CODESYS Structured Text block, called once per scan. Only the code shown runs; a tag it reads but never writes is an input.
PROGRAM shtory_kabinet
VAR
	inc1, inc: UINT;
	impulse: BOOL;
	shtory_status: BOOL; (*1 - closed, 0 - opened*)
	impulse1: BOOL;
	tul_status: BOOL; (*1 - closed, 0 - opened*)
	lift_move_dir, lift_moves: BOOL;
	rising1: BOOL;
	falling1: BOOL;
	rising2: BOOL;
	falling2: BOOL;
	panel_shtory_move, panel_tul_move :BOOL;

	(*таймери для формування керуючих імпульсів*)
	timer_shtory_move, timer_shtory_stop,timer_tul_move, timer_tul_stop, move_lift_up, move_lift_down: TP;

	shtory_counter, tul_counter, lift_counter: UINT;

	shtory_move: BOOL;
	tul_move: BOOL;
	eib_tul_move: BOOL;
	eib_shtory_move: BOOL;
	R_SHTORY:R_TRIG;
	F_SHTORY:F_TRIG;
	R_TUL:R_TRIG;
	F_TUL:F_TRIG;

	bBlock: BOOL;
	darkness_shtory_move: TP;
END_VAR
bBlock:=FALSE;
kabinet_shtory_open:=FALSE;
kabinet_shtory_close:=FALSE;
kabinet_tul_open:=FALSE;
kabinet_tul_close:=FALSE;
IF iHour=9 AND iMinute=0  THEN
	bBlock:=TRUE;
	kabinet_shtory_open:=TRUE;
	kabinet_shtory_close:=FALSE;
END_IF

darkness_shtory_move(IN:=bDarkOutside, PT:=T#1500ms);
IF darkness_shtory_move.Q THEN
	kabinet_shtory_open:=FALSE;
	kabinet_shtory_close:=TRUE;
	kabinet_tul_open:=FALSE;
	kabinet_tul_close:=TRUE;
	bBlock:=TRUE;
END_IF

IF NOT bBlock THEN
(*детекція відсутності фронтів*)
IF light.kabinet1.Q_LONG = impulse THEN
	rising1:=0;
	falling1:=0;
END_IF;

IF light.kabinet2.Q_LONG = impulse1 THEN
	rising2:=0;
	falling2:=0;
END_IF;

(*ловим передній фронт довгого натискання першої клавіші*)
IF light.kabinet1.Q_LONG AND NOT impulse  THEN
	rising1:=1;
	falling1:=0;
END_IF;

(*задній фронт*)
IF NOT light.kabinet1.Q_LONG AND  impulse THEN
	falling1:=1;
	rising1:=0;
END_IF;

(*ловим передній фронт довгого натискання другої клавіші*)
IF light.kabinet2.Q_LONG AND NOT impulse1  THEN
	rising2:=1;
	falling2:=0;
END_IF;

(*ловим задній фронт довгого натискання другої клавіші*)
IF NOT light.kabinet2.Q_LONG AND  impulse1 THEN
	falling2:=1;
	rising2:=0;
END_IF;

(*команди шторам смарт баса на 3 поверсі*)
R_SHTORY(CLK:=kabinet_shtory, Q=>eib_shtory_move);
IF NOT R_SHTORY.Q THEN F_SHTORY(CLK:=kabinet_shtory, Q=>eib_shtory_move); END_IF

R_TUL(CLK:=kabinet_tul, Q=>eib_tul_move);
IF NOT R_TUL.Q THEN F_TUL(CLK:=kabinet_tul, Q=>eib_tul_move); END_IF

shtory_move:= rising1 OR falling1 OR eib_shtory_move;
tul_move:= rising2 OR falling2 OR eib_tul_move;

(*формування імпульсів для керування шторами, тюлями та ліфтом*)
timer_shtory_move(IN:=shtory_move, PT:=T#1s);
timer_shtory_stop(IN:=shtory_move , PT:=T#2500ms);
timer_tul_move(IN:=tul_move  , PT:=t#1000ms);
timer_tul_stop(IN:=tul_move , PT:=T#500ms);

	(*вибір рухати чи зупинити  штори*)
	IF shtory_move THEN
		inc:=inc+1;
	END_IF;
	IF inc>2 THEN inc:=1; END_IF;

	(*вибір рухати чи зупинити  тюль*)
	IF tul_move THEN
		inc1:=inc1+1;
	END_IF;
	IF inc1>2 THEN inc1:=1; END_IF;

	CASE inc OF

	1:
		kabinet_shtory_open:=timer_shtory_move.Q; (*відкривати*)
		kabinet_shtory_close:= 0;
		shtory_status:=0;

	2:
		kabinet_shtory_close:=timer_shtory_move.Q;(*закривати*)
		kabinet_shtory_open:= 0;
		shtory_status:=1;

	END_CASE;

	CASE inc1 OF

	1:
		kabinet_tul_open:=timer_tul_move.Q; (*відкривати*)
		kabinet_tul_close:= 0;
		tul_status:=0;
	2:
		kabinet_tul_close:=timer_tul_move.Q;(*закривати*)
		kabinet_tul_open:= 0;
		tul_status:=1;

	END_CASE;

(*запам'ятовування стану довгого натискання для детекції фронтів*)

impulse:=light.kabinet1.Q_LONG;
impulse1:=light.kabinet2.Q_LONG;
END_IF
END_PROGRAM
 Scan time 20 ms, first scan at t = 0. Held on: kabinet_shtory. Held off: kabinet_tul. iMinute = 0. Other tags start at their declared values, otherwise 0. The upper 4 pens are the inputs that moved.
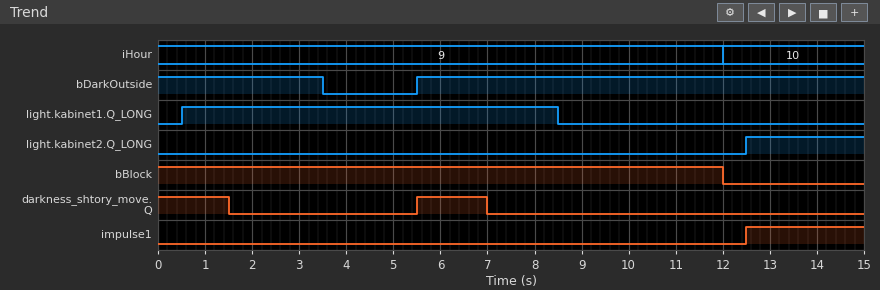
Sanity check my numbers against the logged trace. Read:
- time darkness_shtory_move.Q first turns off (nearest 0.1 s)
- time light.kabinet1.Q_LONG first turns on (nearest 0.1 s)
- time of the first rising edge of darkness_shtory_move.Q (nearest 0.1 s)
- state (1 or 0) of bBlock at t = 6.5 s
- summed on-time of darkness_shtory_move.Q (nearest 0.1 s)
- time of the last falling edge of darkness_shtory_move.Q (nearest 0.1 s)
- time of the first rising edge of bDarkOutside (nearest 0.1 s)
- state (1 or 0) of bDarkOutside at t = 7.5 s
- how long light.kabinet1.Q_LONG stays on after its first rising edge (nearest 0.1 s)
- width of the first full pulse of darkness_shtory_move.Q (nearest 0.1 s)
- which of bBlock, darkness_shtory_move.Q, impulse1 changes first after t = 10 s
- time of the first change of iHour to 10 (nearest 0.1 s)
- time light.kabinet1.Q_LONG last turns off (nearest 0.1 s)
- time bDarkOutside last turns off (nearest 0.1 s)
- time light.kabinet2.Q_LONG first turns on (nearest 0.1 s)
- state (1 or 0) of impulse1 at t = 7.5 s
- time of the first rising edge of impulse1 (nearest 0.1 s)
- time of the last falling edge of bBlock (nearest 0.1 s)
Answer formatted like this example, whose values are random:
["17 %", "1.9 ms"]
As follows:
["1.5 s", "0.5 s", "5.5 s", "1", "3.0 s", "7.0 s", "5.5 s", "1", "8.0 s", "1.5 s", "bBlock", "12.0 s", "8.5 s", "3.5 s", "12.5 s", "0", "12.5 s", "12.0 s"]
